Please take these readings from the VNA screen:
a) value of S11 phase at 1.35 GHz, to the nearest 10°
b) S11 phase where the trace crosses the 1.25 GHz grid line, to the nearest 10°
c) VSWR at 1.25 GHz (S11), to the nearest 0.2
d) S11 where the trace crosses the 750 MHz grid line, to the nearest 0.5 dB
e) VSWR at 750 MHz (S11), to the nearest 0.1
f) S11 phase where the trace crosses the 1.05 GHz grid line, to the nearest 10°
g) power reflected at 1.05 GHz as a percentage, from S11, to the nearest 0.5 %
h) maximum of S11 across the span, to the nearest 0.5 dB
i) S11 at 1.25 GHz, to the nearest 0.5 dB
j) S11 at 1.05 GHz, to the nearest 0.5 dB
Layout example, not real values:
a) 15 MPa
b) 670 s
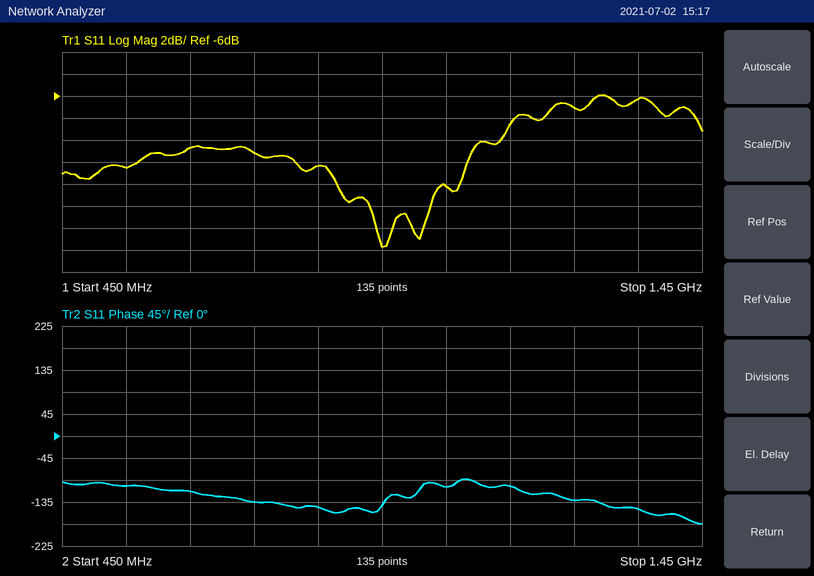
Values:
a) -150°
b) -130°
c) 2.6
d) -11.0 dB
e) 1.8
f) -100°
g) 4.0 %
h) -6.0 dB
i) -7.0 dB
j) -14.0 dB
